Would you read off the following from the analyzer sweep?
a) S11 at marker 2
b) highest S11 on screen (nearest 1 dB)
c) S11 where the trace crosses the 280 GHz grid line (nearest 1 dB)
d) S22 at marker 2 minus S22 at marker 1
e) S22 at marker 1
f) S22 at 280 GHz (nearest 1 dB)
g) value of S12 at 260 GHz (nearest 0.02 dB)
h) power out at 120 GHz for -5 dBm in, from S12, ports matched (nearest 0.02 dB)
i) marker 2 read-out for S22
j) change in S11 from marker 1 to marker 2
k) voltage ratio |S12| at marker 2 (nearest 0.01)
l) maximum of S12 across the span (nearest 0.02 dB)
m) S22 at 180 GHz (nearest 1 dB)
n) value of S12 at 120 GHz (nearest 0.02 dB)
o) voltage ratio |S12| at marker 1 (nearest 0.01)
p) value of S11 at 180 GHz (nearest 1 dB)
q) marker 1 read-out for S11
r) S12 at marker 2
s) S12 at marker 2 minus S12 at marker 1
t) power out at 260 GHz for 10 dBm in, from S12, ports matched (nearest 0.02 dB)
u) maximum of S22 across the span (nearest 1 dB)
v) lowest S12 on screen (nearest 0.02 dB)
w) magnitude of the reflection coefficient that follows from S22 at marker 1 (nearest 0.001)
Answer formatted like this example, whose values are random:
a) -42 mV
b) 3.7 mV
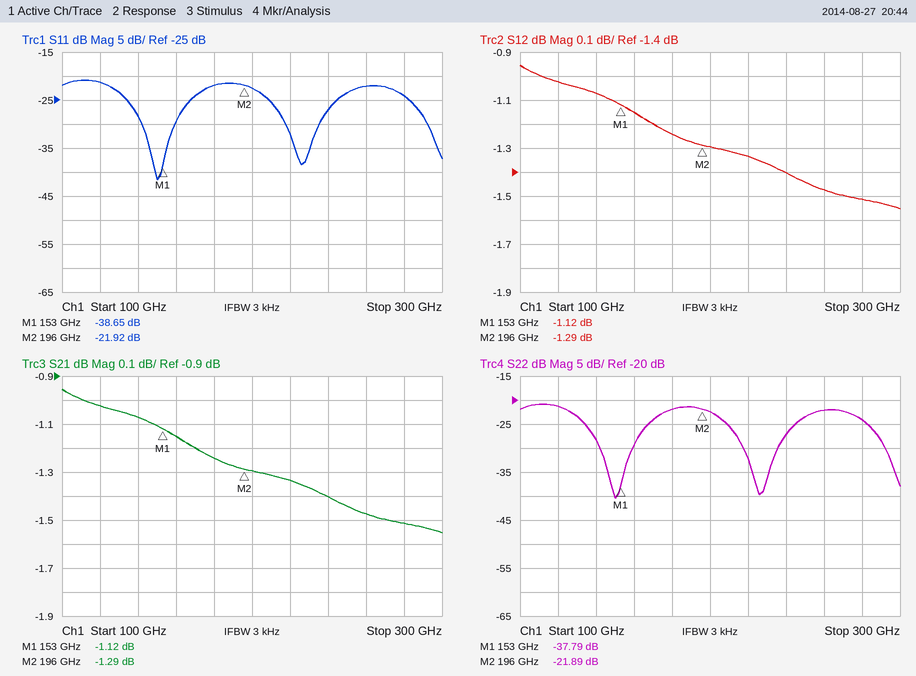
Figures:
a) -21.92 dB
b) -21 dB
c) -24 dB
d) 15.90 dB
e) -37.79 dB
f) -24 dB
g) -1.48 dB
h) -6.02 dBm
i) -21.89 dB
j) 16.73 dB
k) 0.86
l) -0.96 dB
m) -22 dB
n) -1.02 dB
o) 0.88
p) -22 dB
q) -38.65 dB
r) -1.29 dB
s) -0.17 dB
t) 8.52 dBm
u) -21 dB
v) -1.56 dB
w) 0.013
